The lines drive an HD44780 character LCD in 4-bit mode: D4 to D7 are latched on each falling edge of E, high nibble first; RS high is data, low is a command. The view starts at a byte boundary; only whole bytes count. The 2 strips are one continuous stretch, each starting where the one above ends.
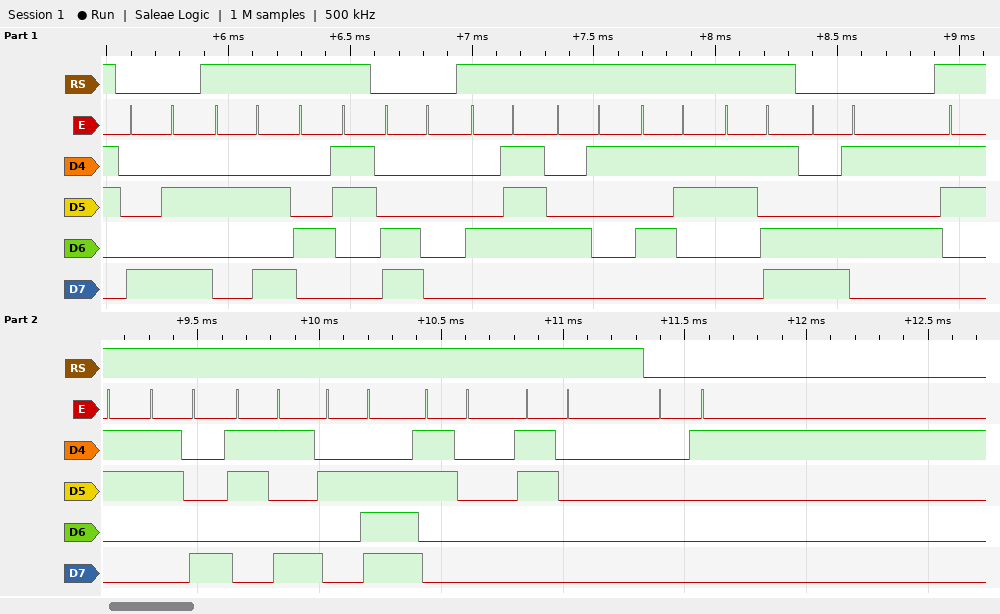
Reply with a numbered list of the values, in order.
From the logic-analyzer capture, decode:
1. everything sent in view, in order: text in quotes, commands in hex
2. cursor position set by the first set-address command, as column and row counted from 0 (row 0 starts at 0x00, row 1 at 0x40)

1. 0x8A "*C" 0xC0 "GAS=" 0xC5 "389.00" 0x01
2. column 10, row 0
